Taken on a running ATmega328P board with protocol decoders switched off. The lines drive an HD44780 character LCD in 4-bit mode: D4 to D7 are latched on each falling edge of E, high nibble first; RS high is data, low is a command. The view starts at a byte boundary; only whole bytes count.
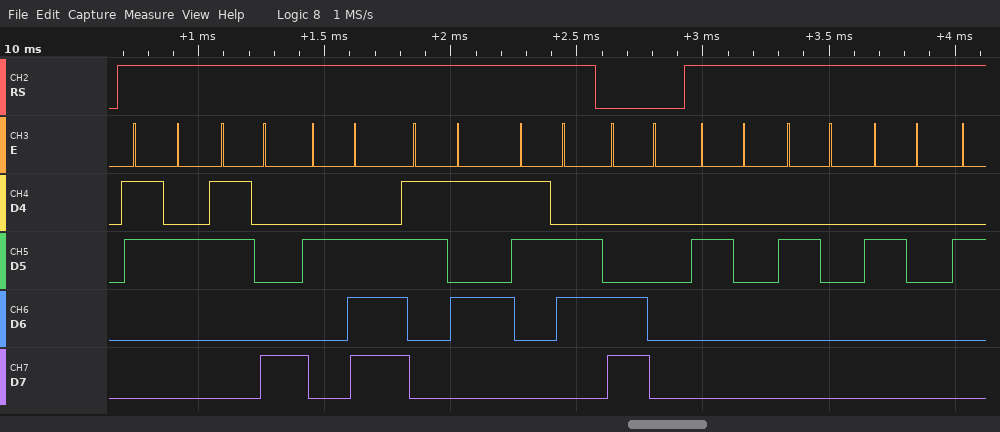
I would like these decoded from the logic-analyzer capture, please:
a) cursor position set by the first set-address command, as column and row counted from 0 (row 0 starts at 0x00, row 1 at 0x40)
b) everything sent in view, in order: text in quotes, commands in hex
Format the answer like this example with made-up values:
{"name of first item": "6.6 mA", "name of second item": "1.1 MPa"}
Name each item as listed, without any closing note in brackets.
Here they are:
{"cursor position set by the first set-address command, as column and row counted from 0": "column 0, row 1", "everything sent in view, in order: text in quotes, commands in hex": "\"28.56\" 0xC0 \"   \""}
